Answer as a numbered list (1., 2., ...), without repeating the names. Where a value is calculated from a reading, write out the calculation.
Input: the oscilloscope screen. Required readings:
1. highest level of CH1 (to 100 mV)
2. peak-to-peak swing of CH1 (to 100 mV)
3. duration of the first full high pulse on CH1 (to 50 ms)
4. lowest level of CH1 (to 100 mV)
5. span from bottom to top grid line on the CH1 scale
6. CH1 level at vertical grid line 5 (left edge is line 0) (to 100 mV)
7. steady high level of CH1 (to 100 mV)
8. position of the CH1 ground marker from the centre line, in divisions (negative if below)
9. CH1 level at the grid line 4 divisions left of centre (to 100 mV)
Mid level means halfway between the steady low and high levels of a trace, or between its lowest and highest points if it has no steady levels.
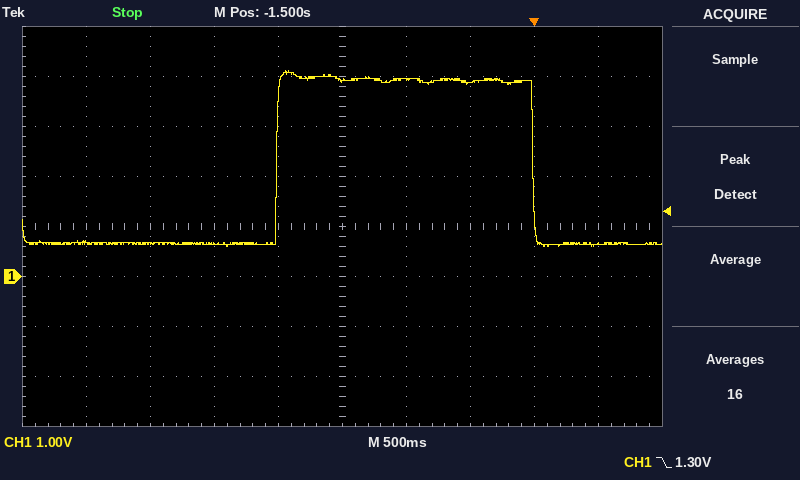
1. 4.1 V
2. 4.1 V − (600 mV) = 3.5 V
3. 2.00 s
4. 600 mV
5. 8 V
6. 3.9 V
7. 3.9 V
8. -1.0 div
9. 700 mV
